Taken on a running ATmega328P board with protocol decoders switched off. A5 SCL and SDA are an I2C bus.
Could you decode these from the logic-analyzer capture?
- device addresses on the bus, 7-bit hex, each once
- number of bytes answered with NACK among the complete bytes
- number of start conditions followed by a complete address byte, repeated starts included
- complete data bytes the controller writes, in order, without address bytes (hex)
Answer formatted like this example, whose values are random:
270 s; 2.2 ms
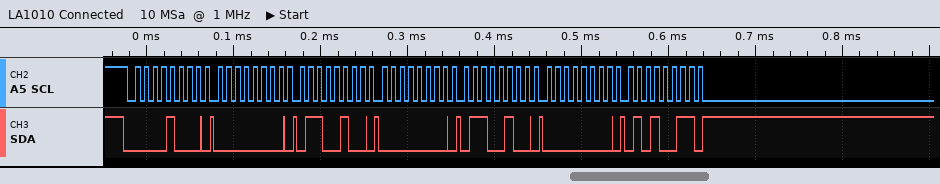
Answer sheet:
0x04; 0; 1; 00 64 00 64 00 53
